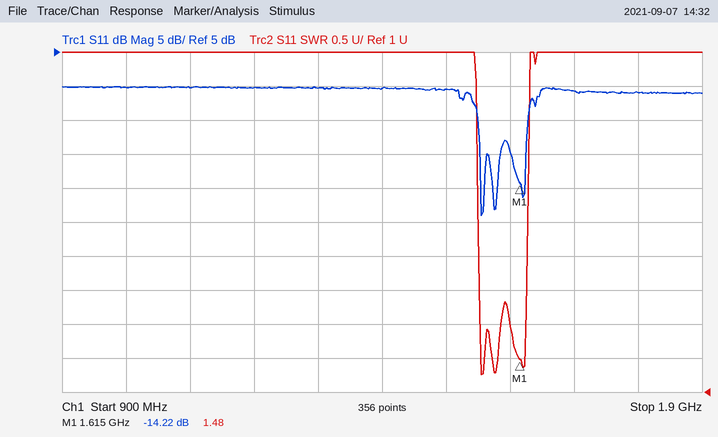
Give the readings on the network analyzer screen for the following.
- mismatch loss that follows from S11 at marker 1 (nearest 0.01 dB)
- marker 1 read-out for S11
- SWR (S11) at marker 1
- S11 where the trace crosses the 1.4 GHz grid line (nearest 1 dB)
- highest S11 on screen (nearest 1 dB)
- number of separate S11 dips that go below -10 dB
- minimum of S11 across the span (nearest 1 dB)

0.17 dB
-14.22 dB
1.48
0 dB
0 dB
3
-19 dB
